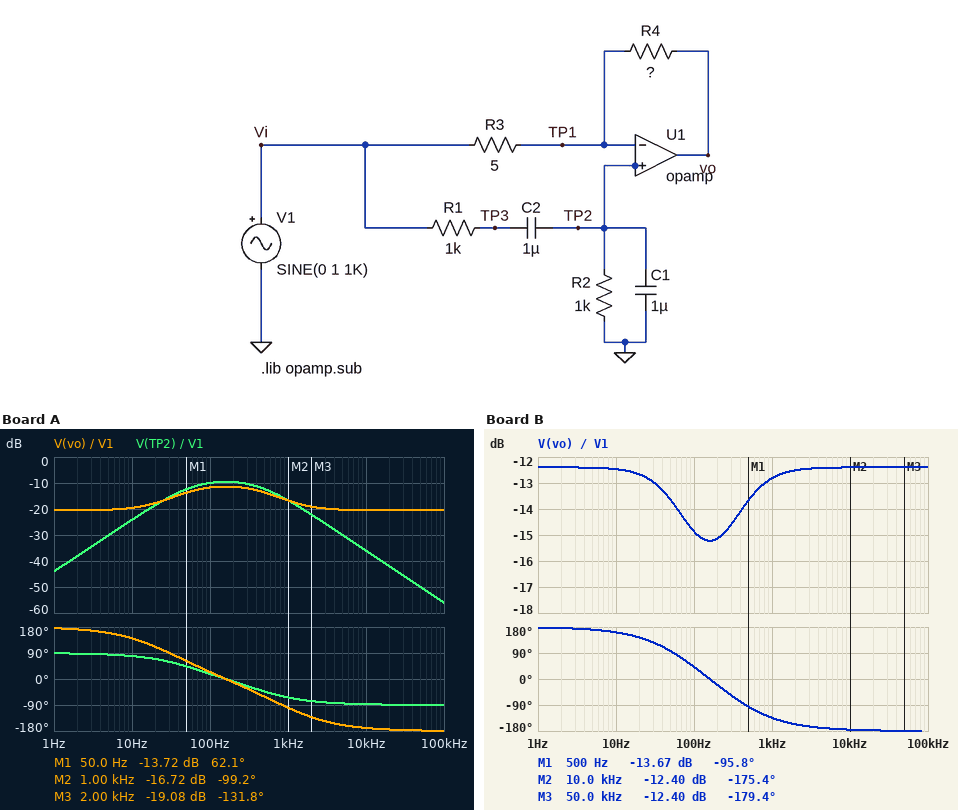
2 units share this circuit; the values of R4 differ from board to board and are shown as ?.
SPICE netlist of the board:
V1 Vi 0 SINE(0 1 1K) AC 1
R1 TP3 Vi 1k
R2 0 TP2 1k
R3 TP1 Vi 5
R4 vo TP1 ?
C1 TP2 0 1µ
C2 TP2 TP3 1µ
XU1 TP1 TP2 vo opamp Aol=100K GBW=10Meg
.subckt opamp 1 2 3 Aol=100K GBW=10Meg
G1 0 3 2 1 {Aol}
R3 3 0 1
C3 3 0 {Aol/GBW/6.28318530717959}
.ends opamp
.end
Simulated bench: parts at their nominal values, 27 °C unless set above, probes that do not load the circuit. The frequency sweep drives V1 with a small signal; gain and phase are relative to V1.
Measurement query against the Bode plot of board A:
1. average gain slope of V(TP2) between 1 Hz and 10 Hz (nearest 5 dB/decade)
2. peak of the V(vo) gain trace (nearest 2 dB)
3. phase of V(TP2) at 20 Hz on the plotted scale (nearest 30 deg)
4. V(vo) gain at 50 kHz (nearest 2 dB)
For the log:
20 dB/decade
-12 dB
60 deg
-20 dB
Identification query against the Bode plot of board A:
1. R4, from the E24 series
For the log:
0.47 Ω
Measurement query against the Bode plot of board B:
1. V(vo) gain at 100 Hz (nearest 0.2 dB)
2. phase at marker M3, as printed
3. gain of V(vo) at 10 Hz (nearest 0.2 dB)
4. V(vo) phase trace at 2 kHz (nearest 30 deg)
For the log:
-14.8 dB
-179.4 deg
-12.4 dB
-150 deg
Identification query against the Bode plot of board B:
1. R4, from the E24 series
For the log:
1.2 Ω
